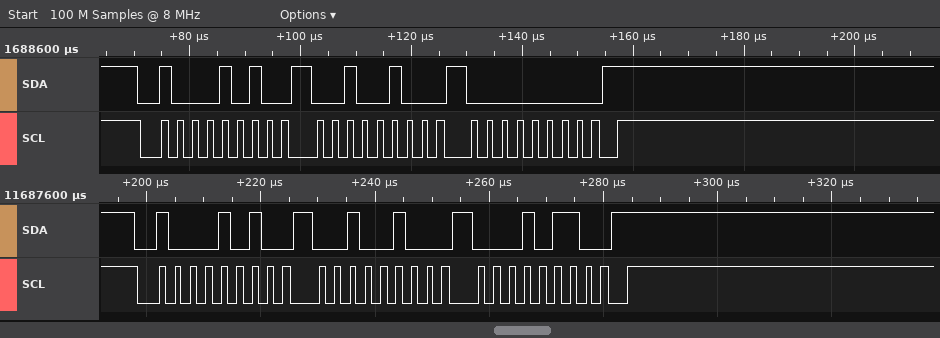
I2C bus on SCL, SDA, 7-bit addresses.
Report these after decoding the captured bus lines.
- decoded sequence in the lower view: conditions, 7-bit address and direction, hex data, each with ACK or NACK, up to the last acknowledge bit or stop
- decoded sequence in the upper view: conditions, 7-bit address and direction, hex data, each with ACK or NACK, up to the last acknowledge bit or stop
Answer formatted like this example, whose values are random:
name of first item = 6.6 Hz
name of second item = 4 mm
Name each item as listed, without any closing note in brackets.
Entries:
decoded sequence in the lower view: conditions, 7-bit address and direction, hex data, each with ACK or NACK, up to the last acknowledge bit or stop = start, address 45 write ACK, 24 ACK, 16 ACK
decoded sequence in the upper view: conditions, 7-bit address and direction, hex data, each with ACK or NACK, up to the last acknowledge bit or stop = start, address 45 write ACK, 24 ACK, 00 ACK
